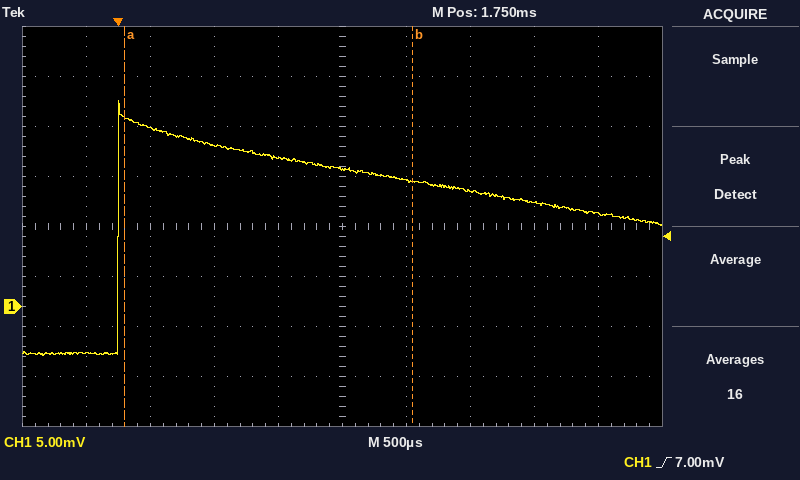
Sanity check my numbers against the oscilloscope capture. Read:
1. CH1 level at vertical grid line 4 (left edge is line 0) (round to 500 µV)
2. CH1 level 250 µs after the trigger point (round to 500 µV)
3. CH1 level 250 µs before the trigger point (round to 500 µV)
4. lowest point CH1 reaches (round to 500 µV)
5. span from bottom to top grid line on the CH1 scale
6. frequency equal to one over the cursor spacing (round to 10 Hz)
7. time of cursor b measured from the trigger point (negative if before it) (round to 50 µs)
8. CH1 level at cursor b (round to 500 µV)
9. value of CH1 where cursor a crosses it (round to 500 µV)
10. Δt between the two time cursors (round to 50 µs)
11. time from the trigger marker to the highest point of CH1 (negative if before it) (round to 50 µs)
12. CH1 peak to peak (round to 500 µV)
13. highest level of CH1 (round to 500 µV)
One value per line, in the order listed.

15.0 mV
18.0 mV
-4.5 mV
-5.0 mV
40 mV
440 Hz
+2.30 ms
12.5 mV
19.0 mV
2.25 ms
0 µs
25.5 mV
20.5 mV
